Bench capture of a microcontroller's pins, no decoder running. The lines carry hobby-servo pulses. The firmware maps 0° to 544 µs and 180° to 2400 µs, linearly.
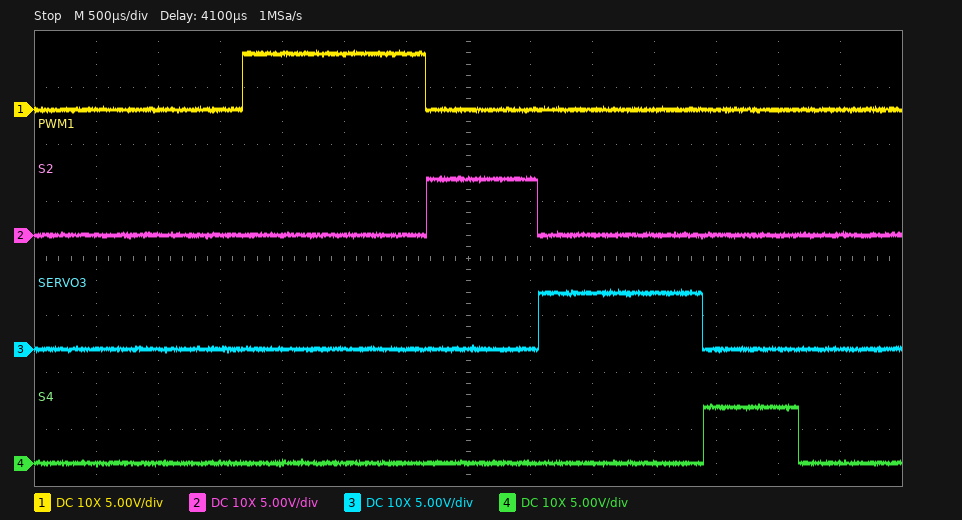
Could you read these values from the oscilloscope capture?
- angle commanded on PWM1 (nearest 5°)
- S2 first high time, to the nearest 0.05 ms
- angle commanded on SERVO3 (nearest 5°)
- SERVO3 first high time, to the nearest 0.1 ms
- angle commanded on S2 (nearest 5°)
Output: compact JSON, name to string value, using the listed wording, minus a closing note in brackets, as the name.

{"angle commanded on PWM1": "90°", "S2 first high time, to the nearest 0.05 ms": "0.90 ms", "angle commanded on SERVO3": "75°", "SERVO3 first high time, to the nearest 0.1 ms": "1.3 ms", "angle commanded on S2": "35°"}
